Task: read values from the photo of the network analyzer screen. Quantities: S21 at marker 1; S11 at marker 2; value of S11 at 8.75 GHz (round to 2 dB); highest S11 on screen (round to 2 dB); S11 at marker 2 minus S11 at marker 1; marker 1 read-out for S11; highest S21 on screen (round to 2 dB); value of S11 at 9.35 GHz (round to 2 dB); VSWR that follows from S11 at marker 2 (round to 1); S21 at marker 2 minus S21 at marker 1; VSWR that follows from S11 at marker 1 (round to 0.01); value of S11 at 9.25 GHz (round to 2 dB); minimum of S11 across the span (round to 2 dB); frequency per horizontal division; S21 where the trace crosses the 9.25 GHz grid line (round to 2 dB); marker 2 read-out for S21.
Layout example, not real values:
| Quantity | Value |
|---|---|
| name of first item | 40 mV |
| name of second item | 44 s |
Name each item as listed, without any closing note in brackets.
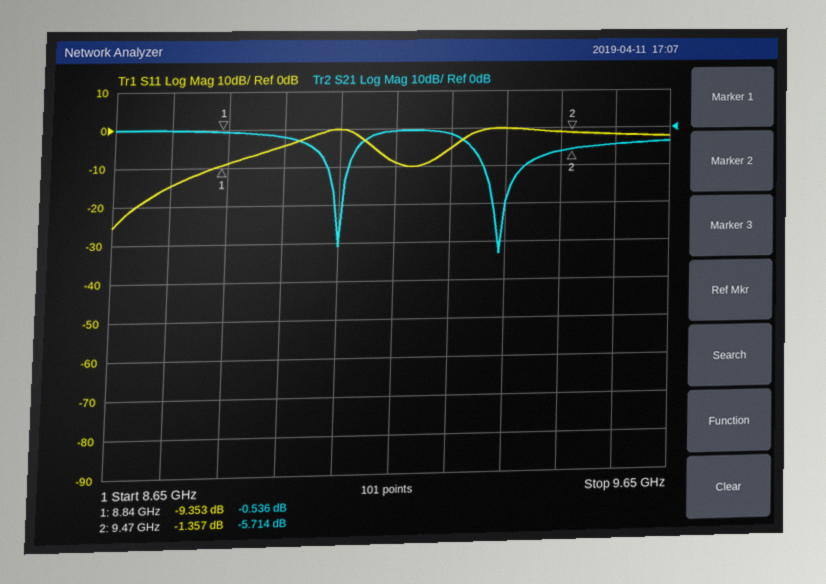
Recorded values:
| Quantity | Value |
|---|---|
| S21 at marker 1 | -0.536 dB |
| S11 at marker 2 | -1.357 dB |
| value of S11 at 8.75 GHz | -14 dB |
| highest S11 on screen | 0 dB |
| S11 at marker 2 minus S11 at marker 1 | 7.996 dB |
| marker 1 read-out for S11 | -9.353 dB |
| highest S21 on screen | 0 dB |
| value of S11 at 9.35 GHz | 0 dB |
| VSWR that follows from S11 at marker 2 | 13 |
| S21 at marker 2 minus S21 at marker 1 | -5.178 dB |
| VSWR that follows from S11 at marker 1 | 2.03 |
| value of S11 at 9.25 GHz | -6 dB |
| minimum of S11 across the span | -26 dB |
| frequency per horizontal division | 100 MHz |
| S21 where the trace crosses the 9.25 GHz grid line | -2 dB |
| marker 2 read-out for S21 | -5.714 dB |
